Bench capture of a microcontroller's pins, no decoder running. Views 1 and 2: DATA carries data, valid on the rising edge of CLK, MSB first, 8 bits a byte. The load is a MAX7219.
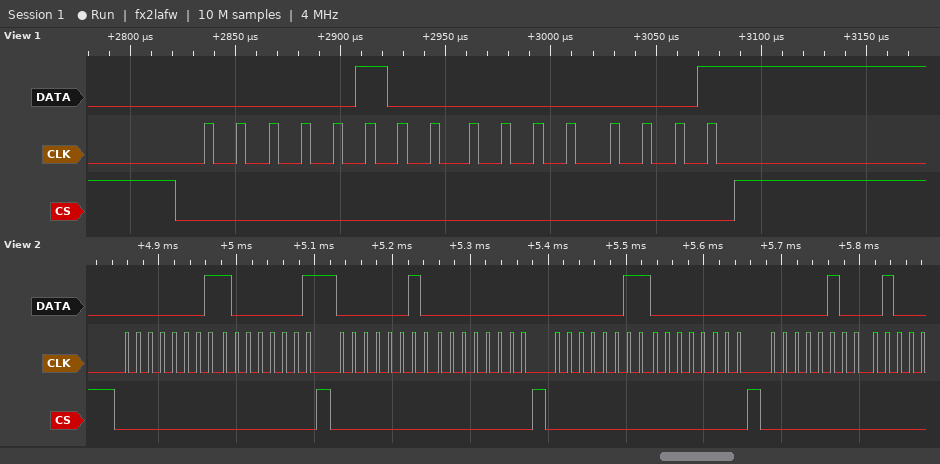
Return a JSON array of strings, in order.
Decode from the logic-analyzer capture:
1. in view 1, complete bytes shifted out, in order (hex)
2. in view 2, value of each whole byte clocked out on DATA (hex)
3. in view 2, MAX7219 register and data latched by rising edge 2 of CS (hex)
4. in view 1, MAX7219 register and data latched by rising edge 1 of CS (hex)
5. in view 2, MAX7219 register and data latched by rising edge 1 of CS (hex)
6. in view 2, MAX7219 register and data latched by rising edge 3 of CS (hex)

["04 01", "01 81 02 00 03 00 04", "register 0x2, data 0x00", "register 0x4, data 0x01", "register 0x1, data 0x81", "register 0x3, data 0x00"]
